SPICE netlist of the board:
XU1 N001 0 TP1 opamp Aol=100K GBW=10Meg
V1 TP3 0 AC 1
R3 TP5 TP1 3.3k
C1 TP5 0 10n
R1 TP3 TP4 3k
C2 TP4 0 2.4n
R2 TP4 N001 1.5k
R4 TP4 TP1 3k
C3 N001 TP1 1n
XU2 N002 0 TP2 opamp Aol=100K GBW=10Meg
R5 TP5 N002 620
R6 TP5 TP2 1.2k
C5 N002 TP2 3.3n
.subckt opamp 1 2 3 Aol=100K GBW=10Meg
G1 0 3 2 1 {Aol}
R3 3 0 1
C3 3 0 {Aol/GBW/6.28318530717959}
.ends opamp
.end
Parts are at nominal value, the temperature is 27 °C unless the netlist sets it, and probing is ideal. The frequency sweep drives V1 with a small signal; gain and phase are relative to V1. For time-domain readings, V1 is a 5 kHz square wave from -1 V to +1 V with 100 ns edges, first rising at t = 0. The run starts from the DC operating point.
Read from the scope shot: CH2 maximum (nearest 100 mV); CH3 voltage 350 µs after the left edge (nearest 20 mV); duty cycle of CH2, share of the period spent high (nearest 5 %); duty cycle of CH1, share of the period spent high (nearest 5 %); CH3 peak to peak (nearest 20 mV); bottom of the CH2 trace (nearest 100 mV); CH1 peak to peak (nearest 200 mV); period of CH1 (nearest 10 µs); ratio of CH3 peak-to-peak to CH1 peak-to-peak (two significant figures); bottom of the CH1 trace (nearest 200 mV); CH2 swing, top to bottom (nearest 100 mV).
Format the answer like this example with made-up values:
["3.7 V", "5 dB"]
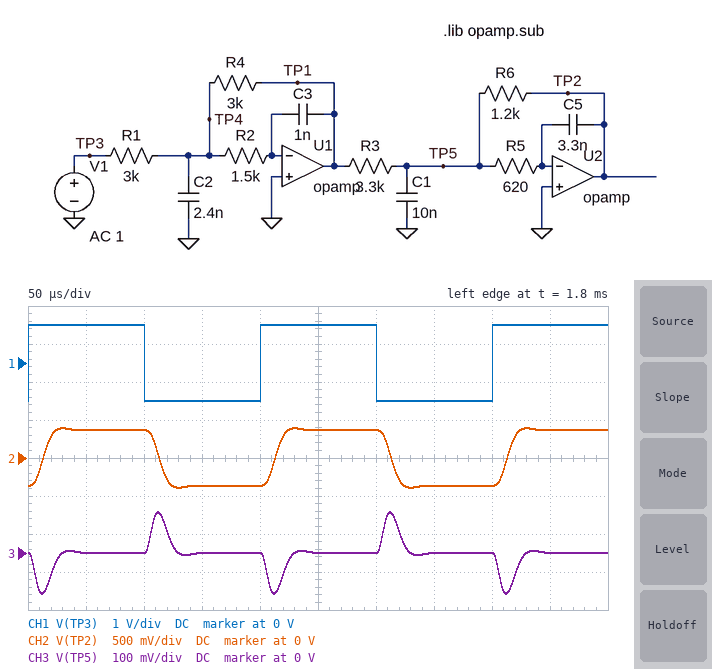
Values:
["400 mV", "0 V", "50 %", "50 %", "220 mV", "-400 mV", "2.0 V", "200 µs", "0.11", "-1.0 V", "800 mV"]
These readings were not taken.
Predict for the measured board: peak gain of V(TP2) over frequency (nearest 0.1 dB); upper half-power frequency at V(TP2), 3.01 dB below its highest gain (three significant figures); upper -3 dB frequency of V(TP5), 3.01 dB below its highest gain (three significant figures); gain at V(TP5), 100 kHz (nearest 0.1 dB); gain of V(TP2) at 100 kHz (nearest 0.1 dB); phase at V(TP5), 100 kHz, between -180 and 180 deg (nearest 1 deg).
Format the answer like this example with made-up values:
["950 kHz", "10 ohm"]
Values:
["-8.8 dB", "26.3 kHz", "43.0 kHz", "-40.3 dB", "-42.6 dB", "-16 deg"]
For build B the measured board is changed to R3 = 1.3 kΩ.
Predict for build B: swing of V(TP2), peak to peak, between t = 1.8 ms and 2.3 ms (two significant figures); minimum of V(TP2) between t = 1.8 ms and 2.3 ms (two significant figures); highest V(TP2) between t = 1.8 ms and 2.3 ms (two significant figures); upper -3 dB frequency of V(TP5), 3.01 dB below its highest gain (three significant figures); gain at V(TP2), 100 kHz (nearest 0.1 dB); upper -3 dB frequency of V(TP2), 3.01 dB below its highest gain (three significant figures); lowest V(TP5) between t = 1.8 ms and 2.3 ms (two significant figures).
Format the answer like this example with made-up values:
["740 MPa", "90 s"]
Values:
["1.9 V", "-940 mV", "940 mV", "43.4 kHz", "-34.8 dB", "22.4 kHz", "-250 mV"]
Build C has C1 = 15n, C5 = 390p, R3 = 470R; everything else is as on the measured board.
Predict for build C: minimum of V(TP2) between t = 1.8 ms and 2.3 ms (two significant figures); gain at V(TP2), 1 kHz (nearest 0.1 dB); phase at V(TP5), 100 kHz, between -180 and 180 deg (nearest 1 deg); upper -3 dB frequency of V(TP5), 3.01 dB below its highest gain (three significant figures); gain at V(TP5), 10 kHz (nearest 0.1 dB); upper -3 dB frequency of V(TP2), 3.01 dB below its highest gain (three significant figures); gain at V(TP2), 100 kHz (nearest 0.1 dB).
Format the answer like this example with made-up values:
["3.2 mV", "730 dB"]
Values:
["-2.7 V", "8.1 dB", "4 deg", "82.9 kHz", "-27.8 dB", "58.3 kHz", "-7.4 dB"]
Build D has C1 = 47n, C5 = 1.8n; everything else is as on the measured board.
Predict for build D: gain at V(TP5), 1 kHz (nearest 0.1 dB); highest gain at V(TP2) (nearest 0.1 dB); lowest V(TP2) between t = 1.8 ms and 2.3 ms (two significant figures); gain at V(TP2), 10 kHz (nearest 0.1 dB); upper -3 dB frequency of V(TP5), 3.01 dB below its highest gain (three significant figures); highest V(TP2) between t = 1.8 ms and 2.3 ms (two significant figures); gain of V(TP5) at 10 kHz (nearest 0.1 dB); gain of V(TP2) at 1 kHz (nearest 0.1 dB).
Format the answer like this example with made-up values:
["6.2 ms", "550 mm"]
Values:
["-51.7 dB", "-2.7 dB", "-660 mV", "-6.9 dB", "24.4 kHz", "660 mV", "-29.9 dB", "-8.8 dB"]
